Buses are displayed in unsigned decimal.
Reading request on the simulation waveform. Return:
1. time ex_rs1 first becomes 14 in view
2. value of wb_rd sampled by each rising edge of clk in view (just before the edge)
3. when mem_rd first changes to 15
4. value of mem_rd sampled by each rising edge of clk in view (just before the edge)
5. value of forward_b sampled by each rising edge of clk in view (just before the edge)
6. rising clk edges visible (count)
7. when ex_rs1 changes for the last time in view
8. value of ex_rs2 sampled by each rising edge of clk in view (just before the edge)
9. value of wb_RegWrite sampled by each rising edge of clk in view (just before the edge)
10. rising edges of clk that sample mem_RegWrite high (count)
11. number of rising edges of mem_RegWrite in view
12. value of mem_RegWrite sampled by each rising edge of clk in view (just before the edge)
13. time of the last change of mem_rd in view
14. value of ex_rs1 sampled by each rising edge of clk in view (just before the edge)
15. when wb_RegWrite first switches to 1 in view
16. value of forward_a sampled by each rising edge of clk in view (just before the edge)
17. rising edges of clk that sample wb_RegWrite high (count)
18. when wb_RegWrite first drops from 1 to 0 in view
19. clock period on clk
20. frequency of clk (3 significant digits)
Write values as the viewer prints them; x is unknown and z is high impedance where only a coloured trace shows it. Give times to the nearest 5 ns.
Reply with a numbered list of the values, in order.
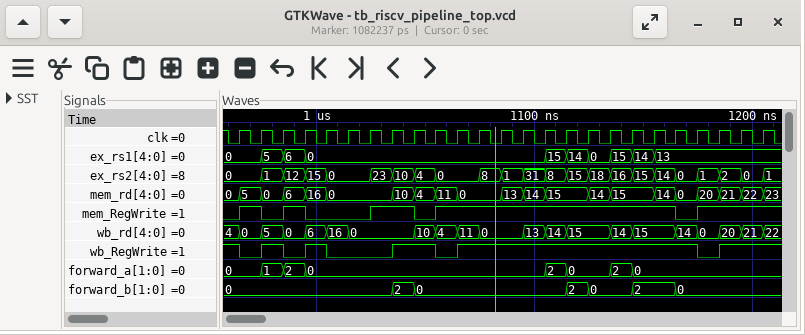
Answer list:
1. 1115 ns
2. 4, 0, 5, 0, 6, 16, 0, 0, 0, 10, 4, 11, 0, 0, 13, 14, 15, 15, 14, 15, 15, 14, 0, 20, 21
3. 1105 ns
4. 0, 5, 0, 6, 16, 0, 0, 0, 10, 4, 11, 0, 0, 13, 14, 15, 15, 14, 15, 15, 14, 0, 20, 21, 22
5. 0, 0, 0, 0, 0, 0, 0, 0, 2, 0, 0, 0, 0, 0, 0, 0, 2, 0, 0, 2, 2, 0, 0, 0, 0
6. 25
7. 1155 ns
8. 0, 0, 1, 12, 15, 0, 0, 23, 10, 4, 0, 0, 8, 1, 31, 8, 15, 18, 16, 15, 14, 0, 1, 2, 0
9. 1 0 1 0 1 0 0 0 1 1 0 1 1 1 1 1 1 1 1 1 1 1 0 1 1
10. 18
11. 5
12. 0 1 0 1 0 0 0 1 1 0 1 1 1 1 1 1 1 1 1 1 1 0 1 1 1
13. 1205 ns
14. 0, 0, 5, 6, 0, 0, 0, 0, 0, 0, 0, 0, 0, 0, 0, 15, 14, 0, 15, 14, 13, 13, 13, 13, 13
15. 975 ns
16. 0, 0, 1, 2, 0, 0, 0, 0, 0, 0, 0, 0, 0, 0, 0, 2, 0, 0, 2, 0, 0, 0, 0, 0, 0
17. 18
18. 965 ns
19. 10 ns
20. 100 MHz
